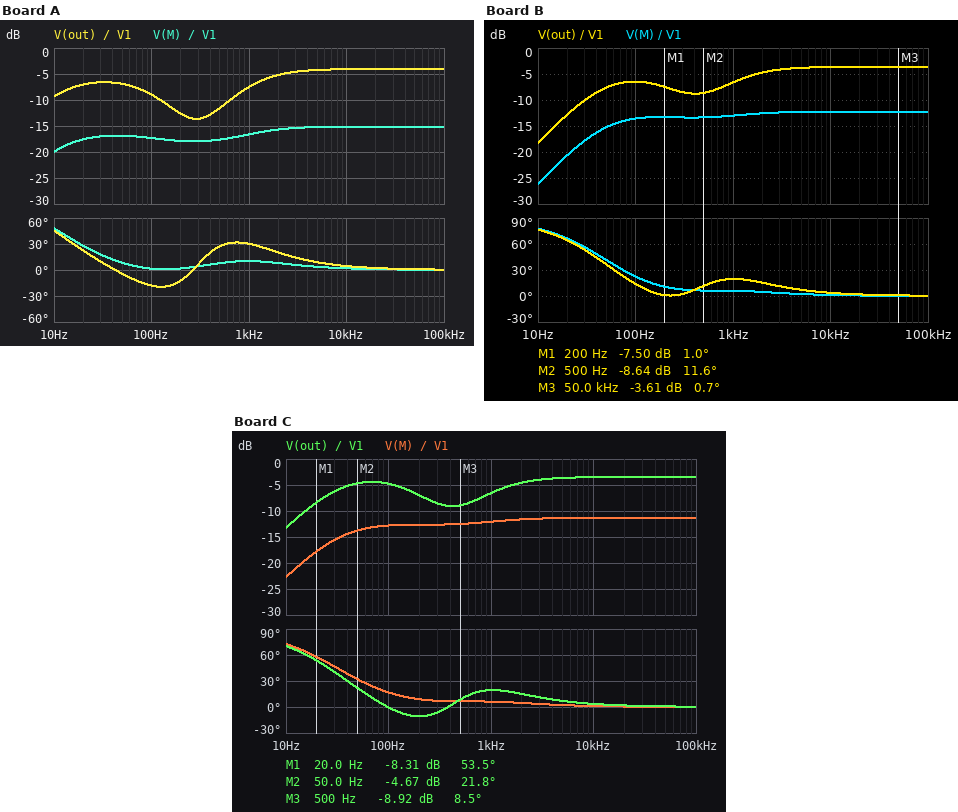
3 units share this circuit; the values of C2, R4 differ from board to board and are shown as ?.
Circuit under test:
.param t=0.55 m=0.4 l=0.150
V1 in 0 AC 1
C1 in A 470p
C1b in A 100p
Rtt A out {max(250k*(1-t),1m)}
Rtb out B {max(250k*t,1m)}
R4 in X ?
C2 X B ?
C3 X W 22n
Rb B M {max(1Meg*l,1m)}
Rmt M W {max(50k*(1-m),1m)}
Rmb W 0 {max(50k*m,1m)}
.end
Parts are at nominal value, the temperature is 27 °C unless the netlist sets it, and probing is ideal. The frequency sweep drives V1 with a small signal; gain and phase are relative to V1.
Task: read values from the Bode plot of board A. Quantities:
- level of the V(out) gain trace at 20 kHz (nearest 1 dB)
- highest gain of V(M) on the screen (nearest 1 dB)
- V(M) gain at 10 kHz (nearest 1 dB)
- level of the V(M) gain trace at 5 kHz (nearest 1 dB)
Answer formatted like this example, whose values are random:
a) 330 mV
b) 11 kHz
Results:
a) -4 dB
b) -15 dB
c) -15 dB
d) -15 dB
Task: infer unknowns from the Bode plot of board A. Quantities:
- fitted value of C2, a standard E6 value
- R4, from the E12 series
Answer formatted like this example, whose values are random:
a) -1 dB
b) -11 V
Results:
a) 33 nF
b) 150 kΩ
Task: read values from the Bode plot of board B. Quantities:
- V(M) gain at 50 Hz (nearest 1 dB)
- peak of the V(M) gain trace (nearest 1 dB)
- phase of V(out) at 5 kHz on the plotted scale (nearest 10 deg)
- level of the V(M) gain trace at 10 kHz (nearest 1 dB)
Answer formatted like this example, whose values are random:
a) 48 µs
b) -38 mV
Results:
a) -15 dB
b) -12 dB
c) 10 deg
d) -12 dB
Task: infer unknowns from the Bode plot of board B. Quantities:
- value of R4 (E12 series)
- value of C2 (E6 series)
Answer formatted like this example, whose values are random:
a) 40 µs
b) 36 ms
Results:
a) 82 kΩ
b) 6.8 nF
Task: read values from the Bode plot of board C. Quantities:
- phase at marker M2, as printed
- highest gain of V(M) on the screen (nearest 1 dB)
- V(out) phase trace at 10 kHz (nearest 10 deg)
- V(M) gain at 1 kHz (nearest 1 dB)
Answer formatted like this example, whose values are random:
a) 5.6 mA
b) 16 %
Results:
a) 21.8 deg
b) -11 dB
c) 0 deg
d) -12 dB
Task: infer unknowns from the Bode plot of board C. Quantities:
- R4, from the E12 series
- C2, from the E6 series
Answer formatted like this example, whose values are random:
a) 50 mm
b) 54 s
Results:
a) 68 kΩ
b) 15 nF
